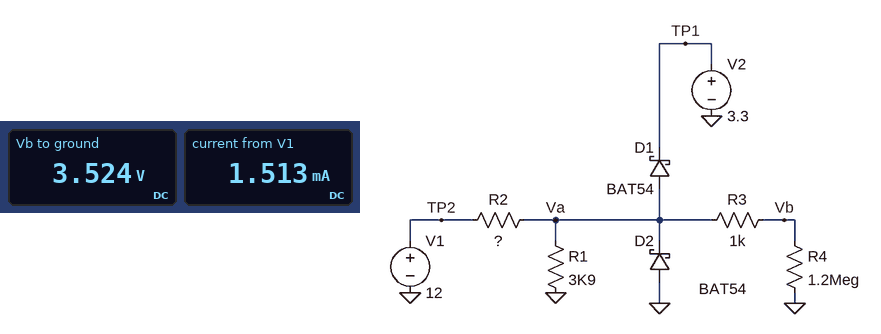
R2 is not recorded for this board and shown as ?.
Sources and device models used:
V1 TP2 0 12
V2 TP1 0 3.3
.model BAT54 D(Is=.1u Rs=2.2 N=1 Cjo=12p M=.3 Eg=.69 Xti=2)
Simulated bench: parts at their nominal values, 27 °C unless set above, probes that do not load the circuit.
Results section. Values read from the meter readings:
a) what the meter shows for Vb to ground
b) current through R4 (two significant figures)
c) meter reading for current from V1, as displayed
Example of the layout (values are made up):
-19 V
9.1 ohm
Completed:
3.524 V
2.9 µA
1.513 mA
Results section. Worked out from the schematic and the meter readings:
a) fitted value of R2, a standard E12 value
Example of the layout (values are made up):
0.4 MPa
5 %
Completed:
5.6 kΩ
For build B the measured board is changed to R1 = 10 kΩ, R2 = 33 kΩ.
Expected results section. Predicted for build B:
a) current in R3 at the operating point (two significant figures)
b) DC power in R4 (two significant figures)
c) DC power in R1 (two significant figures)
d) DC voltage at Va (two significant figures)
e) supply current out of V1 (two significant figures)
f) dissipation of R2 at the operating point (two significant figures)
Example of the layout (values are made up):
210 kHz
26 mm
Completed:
2.3 µA
6.4 µW
770 µW
2.8 V
280 µA
2.6 mW
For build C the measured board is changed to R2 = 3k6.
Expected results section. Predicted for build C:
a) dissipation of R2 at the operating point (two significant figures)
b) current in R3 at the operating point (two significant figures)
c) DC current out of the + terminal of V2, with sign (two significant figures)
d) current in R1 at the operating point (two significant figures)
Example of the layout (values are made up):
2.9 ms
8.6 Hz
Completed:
20 mW
3.0 µA
-1.4 mA
910 µA
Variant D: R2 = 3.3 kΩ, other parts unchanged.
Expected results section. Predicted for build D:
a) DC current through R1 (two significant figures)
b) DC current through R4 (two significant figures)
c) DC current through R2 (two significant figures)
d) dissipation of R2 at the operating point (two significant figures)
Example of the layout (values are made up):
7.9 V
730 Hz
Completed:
910 µA
3.0 µA
2.6 mA
22 mW
